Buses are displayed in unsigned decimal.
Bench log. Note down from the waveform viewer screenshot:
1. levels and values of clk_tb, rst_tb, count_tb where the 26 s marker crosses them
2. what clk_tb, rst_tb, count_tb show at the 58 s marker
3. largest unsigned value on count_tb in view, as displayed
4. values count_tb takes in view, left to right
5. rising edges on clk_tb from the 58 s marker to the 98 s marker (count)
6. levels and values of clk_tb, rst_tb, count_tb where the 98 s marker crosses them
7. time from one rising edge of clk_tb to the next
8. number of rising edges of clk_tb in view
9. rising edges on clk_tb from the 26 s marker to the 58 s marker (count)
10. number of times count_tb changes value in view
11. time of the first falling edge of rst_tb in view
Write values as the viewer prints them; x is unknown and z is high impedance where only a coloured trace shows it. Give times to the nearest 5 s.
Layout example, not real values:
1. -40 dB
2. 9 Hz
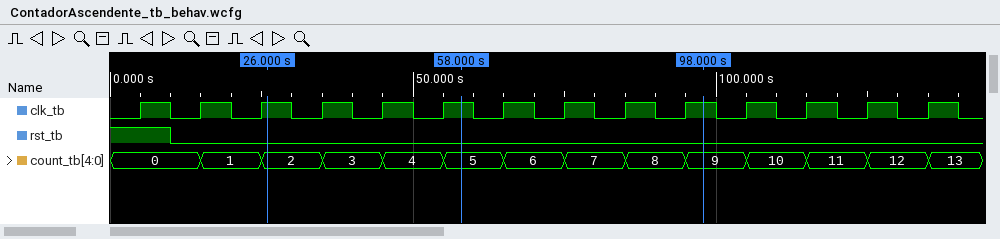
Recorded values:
1. clk_tb=1, rst_tb=0, count_tb=2
2. clk_tb=1, rst_tb=0, count_tb=5
3. 13
4. 0, 1, 2, 3, 4, 5, 6, 7, 8, 9, 10, 11, 12, 13
5. 4
6. clk_tb=1, rst_tb=0, count_tb=9
7. 10 s
8. 14
9. 3
10. 13
11. 10 s
